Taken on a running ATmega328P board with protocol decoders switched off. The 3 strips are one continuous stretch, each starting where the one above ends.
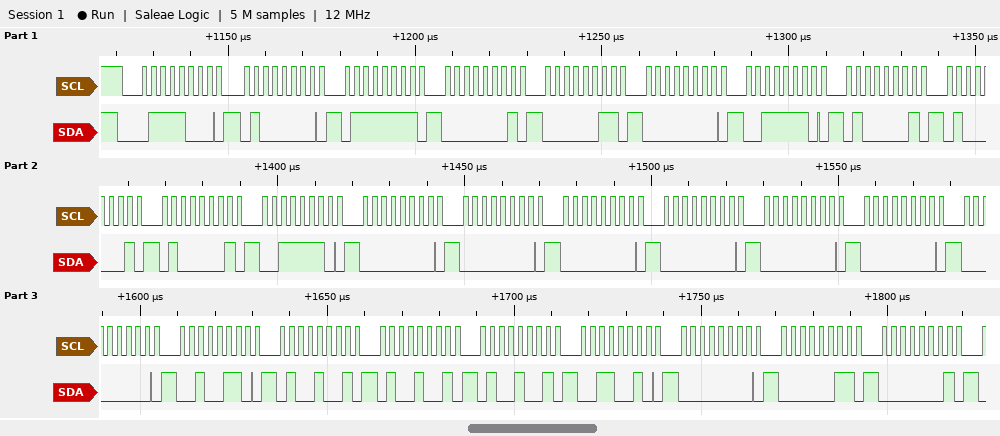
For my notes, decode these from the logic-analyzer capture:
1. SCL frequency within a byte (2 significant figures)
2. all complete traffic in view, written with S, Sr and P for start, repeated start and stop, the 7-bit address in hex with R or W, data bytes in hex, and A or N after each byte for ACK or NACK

400 kHz
S 3CW A 40 A 7F A 01 A 03 A 00 A 3E A 41 A 41 A 41 A 3E A 00 A 00 A 00 A 00 A 00 A 00 A 00 A 26 A 49 A 49 A 49 A 32 A 00 A 03 A 01 A
